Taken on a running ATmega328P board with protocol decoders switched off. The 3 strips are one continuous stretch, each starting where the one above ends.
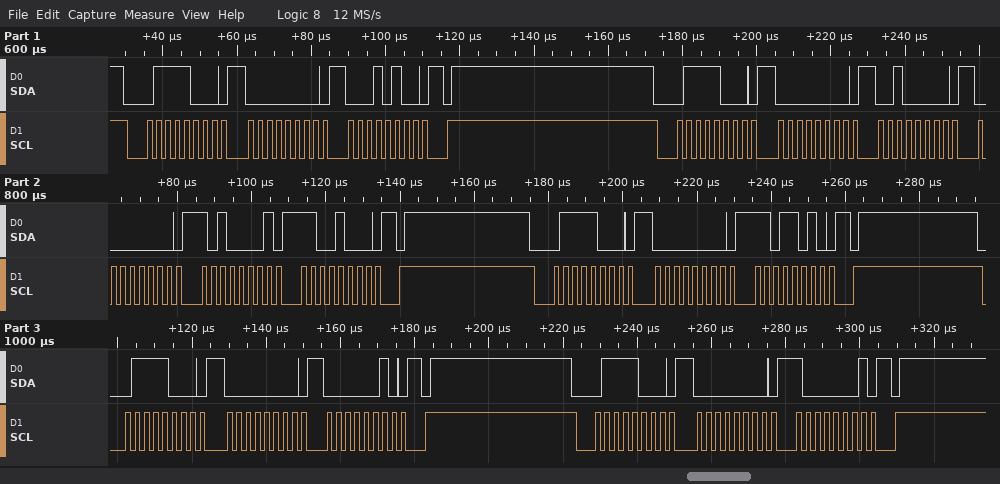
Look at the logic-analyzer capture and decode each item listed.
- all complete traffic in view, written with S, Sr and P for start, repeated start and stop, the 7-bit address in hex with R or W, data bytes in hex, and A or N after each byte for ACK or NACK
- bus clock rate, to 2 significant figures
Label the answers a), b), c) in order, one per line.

a) S 3CW A 00 A 14 A P S 3CW A 00 A 20 A 00 A A1 A C8 A P S 3CW A 00 A DA A P S 3CW A 00 A 02 A P S 3CW A 00 A 81 A P
b) 400 kHz
